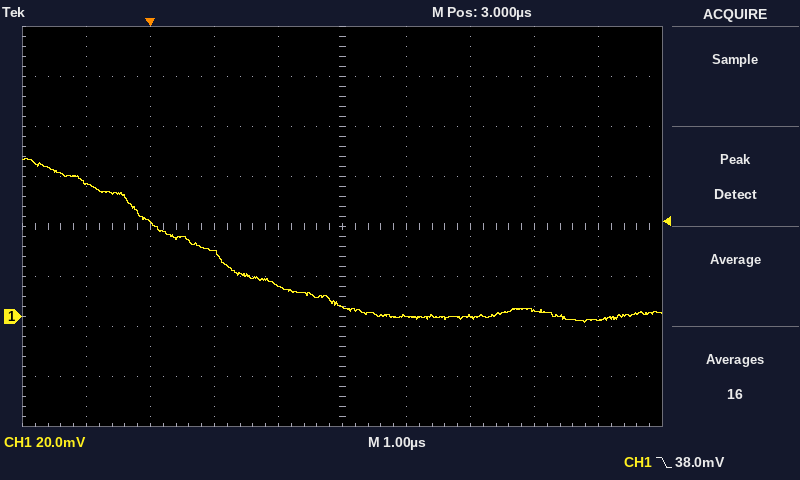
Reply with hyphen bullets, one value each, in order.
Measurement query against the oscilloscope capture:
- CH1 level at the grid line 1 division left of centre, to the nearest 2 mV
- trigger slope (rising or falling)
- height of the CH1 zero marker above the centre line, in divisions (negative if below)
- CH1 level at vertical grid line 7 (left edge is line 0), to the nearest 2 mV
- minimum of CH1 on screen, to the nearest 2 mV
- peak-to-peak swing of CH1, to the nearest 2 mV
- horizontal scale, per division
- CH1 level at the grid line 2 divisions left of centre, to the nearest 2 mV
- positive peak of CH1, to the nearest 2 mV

- 12 mV
- falling
- -1.8 div
- 0 mV
- -2 mV
- 66 mV
- 1 µs
- 26 mV
- 64 mV
